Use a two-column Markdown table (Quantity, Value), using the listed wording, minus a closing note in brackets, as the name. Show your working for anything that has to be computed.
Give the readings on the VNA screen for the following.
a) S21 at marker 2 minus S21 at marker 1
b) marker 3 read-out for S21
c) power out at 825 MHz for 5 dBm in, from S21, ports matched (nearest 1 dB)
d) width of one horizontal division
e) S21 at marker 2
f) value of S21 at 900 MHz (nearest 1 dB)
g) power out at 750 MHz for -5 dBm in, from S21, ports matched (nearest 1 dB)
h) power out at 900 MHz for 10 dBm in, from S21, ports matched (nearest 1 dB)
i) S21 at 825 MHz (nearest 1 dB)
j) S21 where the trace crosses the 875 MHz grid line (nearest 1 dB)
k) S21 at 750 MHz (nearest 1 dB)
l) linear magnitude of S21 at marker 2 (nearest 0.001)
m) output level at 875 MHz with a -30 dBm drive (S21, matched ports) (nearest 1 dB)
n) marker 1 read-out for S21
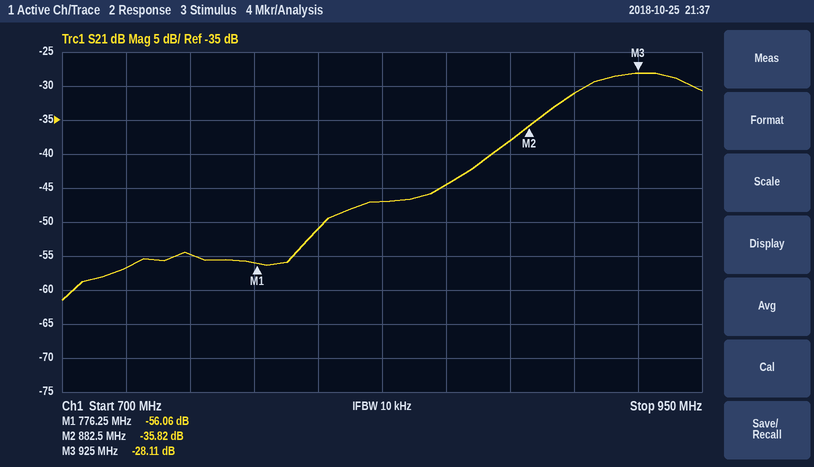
| Quantity | Value |
|---|---|
| S21 at marker 2 minus S21 at marker 1 | -35.82 − (-56.06) = 20.24 dB |
| marker 3 read-out for S21 | -28.11 dB |
| power out at 825 MHz for 5 dBm in, from S21, ports matched | 5 dBm + (-47 dB) = -42 dBm |
| width of one horizontal division | 25 MHz |
| S21 at marker 2 | -35.82 dB |
| value of S21 at 900 MHz | -31 dB |
| power out at 750 MHz for -5 dBm in, from S21, ports matched | -5 dBm + (-55 dB) = -60 dBm |
| power out at 900 MHz for 10 dBm in, from S21, ports matched | 10 dBm + (-31 dB) = -21 dBm |
| S21 at 825 MHz | -47 dB |
| S21 where the trace crosses the 875 MHz grid line | -38 dB |
| S21 at 750 MHz | -55 dB |
| linear magnitude of S21 at marker 2 | 10^(-35.82/20) ≈ 0.016 |
| output level at 875 MHz with a -30 dBm drive (S21, matched ports) | -30 dBm + (-38 dB) = -68 dBm |
| marker 1 read-out for S21 | -56.06 dB |
